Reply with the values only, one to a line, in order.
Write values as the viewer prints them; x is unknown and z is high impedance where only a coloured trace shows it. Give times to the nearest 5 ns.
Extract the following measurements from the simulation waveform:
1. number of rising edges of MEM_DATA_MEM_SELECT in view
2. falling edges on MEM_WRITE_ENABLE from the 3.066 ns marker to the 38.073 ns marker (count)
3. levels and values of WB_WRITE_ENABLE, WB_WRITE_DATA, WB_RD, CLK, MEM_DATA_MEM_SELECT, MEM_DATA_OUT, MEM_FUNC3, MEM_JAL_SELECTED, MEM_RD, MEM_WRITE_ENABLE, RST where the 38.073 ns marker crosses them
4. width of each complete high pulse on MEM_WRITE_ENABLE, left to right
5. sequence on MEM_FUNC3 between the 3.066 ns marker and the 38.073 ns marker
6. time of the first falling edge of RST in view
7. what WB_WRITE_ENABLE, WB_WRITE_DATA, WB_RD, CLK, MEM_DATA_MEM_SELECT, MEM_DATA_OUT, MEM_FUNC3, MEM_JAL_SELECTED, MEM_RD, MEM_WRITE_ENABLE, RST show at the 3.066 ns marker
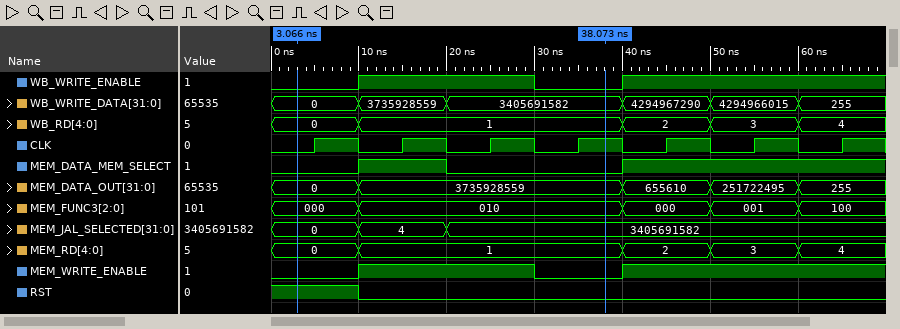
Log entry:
2
1
WB_WRITE_ENABLE=0, WB_WRITE_DATA=3405691582, WB_RD=1, CLK=1, MEM_DATA_MEM_SELECT=0, MEM_DATA_OUT=3735928559, MEM_FUNC3=010, MEM_JAL_SELECTED=3405691582, MEM_RD=1, MEM_WRITE_ENABLE=0, RST=0
20 ns
000, 010
10 ns
WB_WRITE_ENABLE=0, WB_WRITE_DATA=0, WB_RD=0, CLK=0, MEM_DATA_MEM_SELECT=0, MEM_DATA_OUT=0, MEM_FUNC3=000, MEM_JAL_SELECTED=0, MEM_RD=0, MEM_WRITE_ENABLE=0, RST=1
